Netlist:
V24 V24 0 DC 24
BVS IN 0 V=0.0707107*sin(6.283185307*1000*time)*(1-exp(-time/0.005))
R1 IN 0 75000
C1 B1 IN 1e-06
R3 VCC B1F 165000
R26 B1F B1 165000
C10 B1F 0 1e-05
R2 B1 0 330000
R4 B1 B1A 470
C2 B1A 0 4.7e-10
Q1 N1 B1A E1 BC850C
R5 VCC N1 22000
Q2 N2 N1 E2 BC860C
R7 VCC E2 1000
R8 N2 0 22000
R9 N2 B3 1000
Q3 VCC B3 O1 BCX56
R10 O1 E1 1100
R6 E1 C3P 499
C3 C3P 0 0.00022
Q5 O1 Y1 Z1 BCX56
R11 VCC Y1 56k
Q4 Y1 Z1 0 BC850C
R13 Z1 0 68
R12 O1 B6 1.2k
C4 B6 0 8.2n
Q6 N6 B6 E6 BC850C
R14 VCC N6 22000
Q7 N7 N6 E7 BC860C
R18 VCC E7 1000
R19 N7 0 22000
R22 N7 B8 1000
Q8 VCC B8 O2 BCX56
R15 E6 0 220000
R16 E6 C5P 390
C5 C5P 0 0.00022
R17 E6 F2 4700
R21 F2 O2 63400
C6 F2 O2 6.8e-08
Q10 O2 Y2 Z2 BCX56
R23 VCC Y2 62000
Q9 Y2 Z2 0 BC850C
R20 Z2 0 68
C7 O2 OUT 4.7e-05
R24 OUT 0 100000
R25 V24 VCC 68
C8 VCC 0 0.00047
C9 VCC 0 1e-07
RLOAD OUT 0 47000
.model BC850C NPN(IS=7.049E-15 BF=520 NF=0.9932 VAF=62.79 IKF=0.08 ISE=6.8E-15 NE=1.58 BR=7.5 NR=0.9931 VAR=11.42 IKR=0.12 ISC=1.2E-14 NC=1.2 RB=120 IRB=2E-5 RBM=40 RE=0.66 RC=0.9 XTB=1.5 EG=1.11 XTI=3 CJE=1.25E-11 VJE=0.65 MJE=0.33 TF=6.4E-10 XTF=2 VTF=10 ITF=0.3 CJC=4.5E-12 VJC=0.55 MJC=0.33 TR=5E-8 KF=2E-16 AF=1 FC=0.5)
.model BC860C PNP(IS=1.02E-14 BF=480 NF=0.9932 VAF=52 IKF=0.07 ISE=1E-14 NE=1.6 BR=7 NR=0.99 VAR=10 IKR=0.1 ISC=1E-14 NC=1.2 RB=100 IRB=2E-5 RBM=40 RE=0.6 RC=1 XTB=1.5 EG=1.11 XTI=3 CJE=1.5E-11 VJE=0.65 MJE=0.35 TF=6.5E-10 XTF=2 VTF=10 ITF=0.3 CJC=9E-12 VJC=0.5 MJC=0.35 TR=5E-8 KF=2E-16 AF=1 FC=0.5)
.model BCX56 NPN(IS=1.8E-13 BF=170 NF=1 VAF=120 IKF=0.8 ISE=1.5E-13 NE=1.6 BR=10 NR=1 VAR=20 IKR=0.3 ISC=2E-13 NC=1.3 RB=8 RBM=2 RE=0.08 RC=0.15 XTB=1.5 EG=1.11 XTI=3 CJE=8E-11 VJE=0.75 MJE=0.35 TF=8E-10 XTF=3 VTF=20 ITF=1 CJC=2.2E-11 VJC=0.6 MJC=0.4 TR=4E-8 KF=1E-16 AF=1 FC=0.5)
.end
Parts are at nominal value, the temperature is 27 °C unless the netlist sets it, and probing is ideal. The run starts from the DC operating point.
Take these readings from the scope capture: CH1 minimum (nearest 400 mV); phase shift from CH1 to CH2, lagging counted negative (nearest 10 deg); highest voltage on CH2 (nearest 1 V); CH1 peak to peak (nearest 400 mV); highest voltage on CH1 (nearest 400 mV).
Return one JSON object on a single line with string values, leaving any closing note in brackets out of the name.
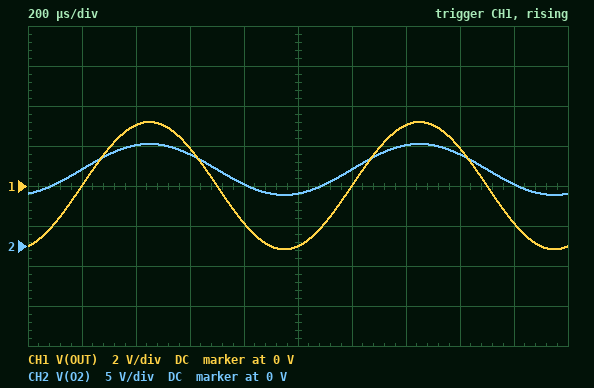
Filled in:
{"CH1 minimum": "-3.2 V", "phase shift from CH1 to CH2, lagging counted negative": "0 deg", "highest voltage on CH2": "13 V", "CH1 peak to peak": "6.4 V", "highest voltage on CH1": "3.2 V"}
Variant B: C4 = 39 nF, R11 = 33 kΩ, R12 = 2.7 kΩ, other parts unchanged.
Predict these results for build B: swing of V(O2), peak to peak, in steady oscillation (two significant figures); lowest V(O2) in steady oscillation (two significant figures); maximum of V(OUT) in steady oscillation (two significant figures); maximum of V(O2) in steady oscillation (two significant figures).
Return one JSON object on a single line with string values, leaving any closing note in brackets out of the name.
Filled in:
{"swing of V(O2), peak to peak, in steady oscillation": "5.3 V", "lowest V(O2) in steady oscillation": "6.9 V", "maximum of V(OUT) in steady oscillation": "2.7 V", "maximum of V(O2) in steady oscillation": "12 V"}
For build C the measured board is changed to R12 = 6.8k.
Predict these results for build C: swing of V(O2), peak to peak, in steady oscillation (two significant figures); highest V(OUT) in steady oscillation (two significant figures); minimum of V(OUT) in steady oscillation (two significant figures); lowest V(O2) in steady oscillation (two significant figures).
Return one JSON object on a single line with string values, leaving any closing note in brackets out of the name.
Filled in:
{"swing of V(O2), peak to peak, in steady oscillation": "6.0 V", "highest V(OUT) in steady oscillation": "3.0 V", "minimum of V(OUT) in steady oscillation": "-3.0 V", "lowest V(O2) in steady oscillation": "6.6 V"}
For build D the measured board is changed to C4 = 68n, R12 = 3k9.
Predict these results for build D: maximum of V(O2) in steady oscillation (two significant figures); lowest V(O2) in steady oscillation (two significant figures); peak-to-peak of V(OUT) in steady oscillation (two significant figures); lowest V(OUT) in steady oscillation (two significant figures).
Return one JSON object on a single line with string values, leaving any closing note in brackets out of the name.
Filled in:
{"maximum of V(O2) in steady oscillation": "11 V", "lowest V(O2) in steady oscillation": "7.9 V", "peak-to-peak of V(OUT) in steady oscillation": "3.3 V", "lowest V(OUT) in steady oscillation": "-1.6 V"}
